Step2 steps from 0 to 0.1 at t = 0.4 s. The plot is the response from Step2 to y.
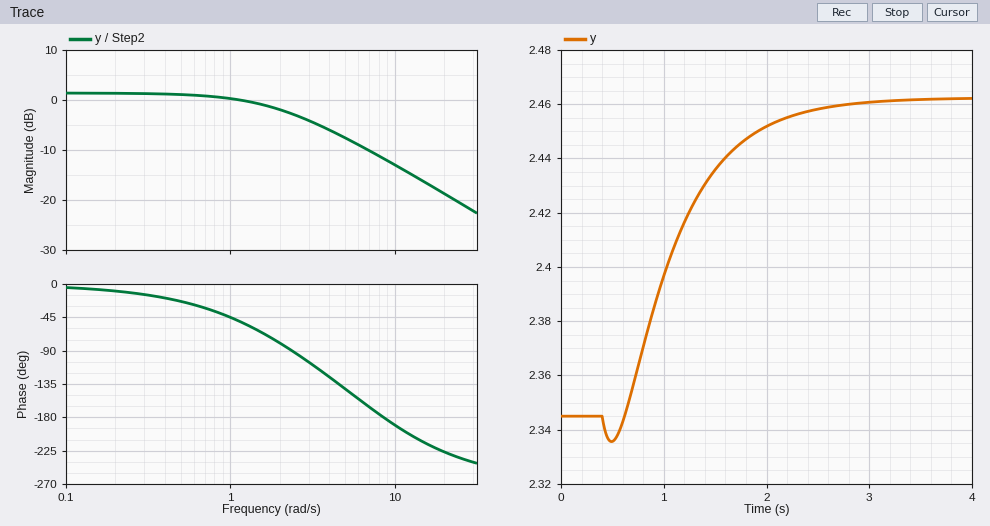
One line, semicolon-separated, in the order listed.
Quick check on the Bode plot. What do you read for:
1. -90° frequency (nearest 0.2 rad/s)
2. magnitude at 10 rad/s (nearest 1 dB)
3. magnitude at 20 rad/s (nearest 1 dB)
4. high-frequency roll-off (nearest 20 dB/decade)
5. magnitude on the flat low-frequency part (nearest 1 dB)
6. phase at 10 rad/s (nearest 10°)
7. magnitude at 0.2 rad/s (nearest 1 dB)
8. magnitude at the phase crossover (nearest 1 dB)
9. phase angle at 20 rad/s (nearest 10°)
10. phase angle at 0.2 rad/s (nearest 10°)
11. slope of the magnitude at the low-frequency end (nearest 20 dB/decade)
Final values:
2.4 rad/s; -13 dB; -19 dB; -20 dB/decade; 1 dB; -190°; 1 dB; -12 dB; -230°; -10°; 0 dB/decade
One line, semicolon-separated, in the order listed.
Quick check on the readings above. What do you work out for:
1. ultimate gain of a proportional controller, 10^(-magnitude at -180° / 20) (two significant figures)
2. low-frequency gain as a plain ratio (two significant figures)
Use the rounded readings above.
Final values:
4.0; 1.1
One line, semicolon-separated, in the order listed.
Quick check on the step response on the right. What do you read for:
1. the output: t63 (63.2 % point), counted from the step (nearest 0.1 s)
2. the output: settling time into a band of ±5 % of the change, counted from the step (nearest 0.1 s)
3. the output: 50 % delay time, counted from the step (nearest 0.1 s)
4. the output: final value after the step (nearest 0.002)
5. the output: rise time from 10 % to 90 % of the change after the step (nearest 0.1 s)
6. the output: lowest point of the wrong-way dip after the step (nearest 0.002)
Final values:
0.8 s; 1.9 s; 0.7 s; 2.462; 1.2 s; 2.336
